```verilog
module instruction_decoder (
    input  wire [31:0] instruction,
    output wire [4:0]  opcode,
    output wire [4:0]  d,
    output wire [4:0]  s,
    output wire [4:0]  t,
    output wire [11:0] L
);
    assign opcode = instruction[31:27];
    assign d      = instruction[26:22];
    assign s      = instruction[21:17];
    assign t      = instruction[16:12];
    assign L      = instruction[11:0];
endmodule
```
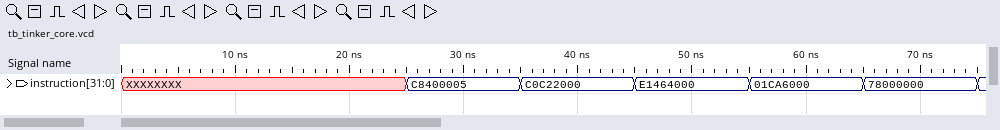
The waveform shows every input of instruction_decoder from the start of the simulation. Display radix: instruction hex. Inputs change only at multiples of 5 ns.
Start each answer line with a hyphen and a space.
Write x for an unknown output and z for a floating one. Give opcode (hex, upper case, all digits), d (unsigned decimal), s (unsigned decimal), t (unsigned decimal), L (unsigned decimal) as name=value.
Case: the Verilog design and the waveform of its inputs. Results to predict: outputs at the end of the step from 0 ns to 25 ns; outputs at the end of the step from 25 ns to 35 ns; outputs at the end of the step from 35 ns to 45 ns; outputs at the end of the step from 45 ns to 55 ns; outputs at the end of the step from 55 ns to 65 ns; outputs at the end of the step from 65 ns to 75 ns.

- opcode=x, d=x, s=x, t=x, L=x
- opcode=19, d=1, s=0, t=0, L=5
- opcode=18, d=3, s=1, t=2, L=0
- opcode=1C, d=5, s=3, t=4, L=0
- opcode=00, d=7, s=5, t=6, L=0
- opcode=0F, d=0, s=0, t=0, L=0
